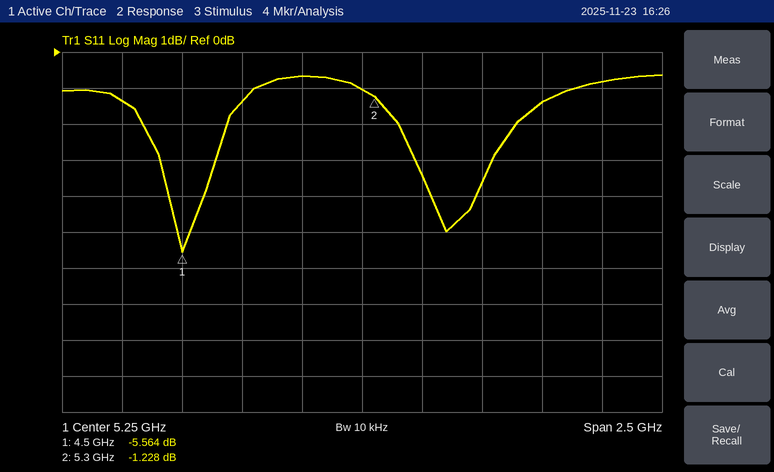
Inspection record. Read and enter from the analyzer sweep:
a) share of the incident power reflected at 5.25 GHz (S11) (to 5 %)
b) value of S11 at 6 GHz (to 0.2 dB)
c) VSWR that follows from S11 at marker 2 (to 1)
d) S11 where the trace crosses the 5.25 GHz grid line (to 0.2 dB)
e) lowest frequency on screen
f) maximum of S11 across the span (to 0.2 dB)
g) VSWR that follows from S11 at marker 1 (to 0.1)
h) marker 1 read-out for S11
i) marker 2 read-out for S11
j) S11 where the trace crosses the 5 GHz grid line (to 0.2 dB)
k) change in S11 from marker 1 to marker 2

80 %
-1.4 dB
14
-1.0 dB
4 GHz
-0.6 dB
3.2
-5.564 dB
-1.228 dB
-0.6 dB
4.336 dB
